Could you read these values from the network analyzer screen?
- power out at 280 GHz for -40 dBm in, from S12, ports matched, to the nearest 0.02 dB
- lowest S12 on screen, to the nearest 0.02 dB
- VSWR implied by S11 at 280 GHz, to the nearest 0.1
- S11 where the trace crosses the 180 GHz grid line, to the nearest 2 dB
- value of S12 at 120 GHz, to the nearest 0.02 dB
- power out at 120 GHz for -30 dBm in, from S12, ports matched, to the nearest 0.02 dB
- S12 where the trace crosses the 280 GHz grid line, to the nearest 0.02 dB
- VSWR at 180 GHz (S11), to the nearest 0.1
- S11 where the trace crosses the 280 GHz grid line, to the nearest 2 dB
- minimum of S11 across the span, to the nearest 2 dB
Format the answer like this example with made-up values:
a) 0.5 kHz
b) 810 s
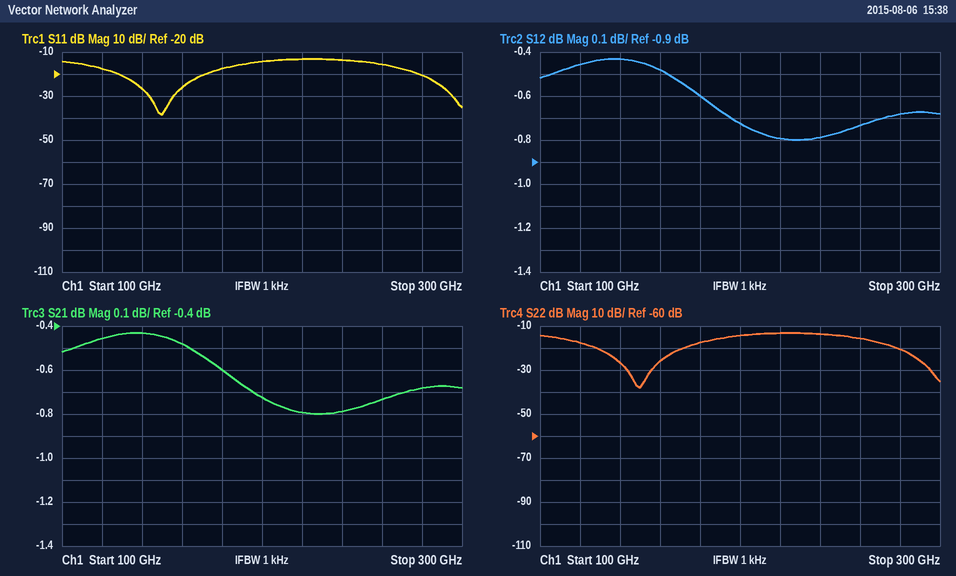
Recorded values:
a) -40.68 dBm
b) -0.80 dB
c) 1.2
d) -18 dB
e) -0.46 dB
f) -30.46 dBm
g) -0.68 dB
h) 1.3
i) -20 dB
j) -38 dB
